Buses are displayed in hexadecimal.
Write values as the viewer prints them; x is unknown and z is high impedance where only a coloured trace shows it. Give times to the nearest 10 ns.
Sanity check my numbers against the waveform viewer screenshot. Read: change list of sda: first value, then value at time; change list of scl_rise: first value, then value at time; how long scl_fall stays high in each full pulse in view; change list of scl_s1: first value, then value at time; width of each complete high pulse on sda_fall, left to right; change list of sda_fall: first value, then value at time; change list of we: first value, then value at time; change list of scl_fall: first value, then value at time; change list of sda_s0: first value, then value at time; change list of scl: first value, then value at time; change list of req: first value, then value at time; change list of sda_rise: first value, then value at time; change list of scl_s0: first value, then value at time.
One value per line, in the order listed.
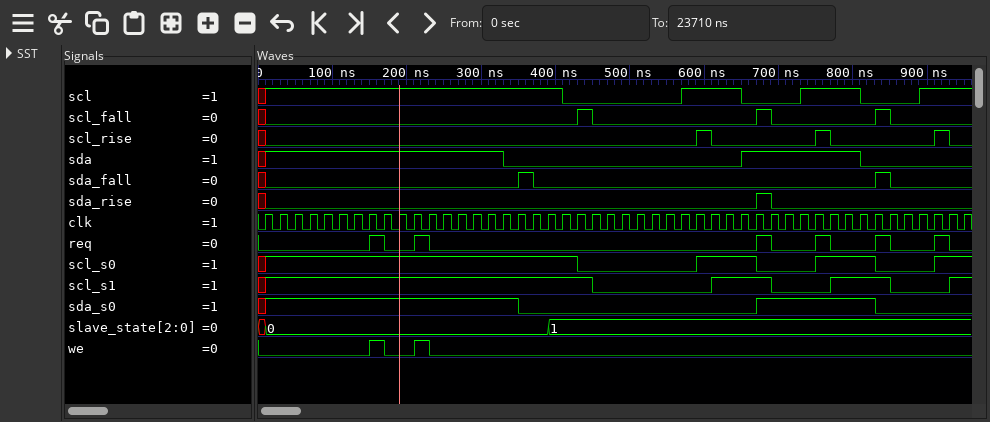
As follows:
x, 1 at 10 ns, 0 at 330 ns, 1 at 650 ns, 0 at 810 ns
x, 0 at 10 ns, 1 at 590 ns, 0 at 610 ns, 1 at 750 ns, 0 at 770 ns, 1 at 910 ns, 0 at 930 ns
20 ns, 20 ns, 20 ns
x, 1 at 10 ns, 0 at 450 ns, 1 at 610 ns, 0 at 690 ns, 1 at 770 ns, 0 at 850 ns, 1 at 930 ns
20 ns, 20 ns
x, 0 at 10 ns, 1 at 350 ns, 0 at 370 ns, 1 at 830 ns, 0 at 850 ns
0, 1 at 150 ns, 0 at 170 ns, 1 at 210 ns, 0 at 230 ns
x, 0 at 10 ns, 1 at 430 ns, 0 at 450 ns, 1 at 670 ns, 0 at 690 ns, 1 at 830 ns, 0 at 850 ns
x, 1 at 10 ns, 0 at 350 ns, 1 at 670 ns, 0 at 830 ns
x, 1 at 10 ns, 0 at 410 ns, 1 at 570 ns, 0 at 650 ns, 1 at 730 ns, 0 at 810 ns, 1 at 890 ns
0, 1 at 150 ns, 0 at 170 ns, 1 at 210 ns, 0 at 230 ns, 1 at 670 ns, 0 at 690 ns, 1 at 750 ns, 0 at 770 ns, 1 at 830 ns, 0 at 850 ns, 1 at 910 ns, 0 at 930 ns
x, 0 at 10 ns, 1 at 670 ns, 0 at 690 ns
x, 1 at 10 ns, 0 at 430 ns, 1 at 590 ns, 0 at 670 ns, 1 at 750 ns, 0 at 830 ns, 1 at 910 ns
